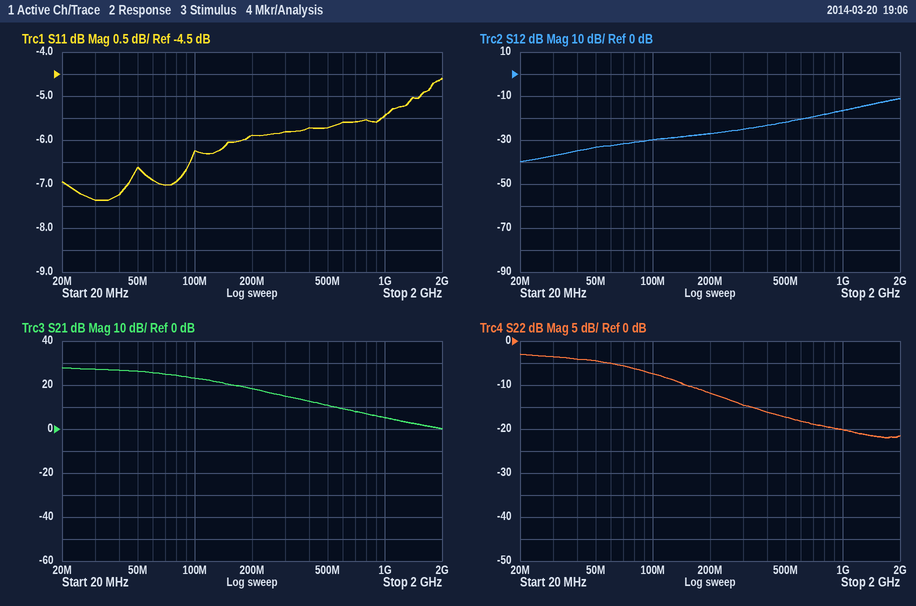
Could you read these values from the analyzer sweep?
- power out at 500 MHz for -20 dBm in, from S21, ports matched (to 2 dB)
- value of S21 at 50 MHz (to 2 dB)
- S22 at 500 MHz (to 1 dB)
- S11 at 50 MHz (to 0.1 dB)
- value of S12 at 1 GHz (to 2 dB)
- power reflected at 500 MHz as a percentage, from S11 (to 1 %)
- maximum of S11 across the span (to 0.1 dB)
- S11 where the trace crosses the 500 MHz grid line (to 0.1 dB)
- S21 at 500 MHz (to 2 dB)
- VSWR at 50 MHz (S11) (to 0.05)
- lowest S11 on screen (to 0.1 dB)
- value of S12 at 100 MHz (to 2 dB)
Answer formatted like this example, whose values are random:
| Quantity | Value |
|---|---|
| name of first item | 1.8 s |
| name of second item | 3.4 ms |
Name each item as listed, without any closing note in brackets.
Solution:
| Quantity | Value |
|---|---|
| power out at 500 MHz for -20 dBm in, from S21, ports matched | -10 dBm |
| value of S21 at 50 MHz | 26 dB |
| S22 at 500 MHz | -17 dB |
| S11 at 50 MHz | -6.6 dB |
| value of S12 at 1 GHz | -16 dB |
| power reflected at 500 MHz as a percentage, from S11 | 27 % |
| maximum of S11 across the span | -4.6 dB |
| S11 where the trace crosses the 500 MHz grid line | -5.7 dB |
| S21 at 500 MHz | 10 dB |
| VSWR at 50 MHz (S11) | 2.75 |
| lowest S11 on screen | -7.4 dB |
| value of S12 at 100 MHz | -30 dB |
